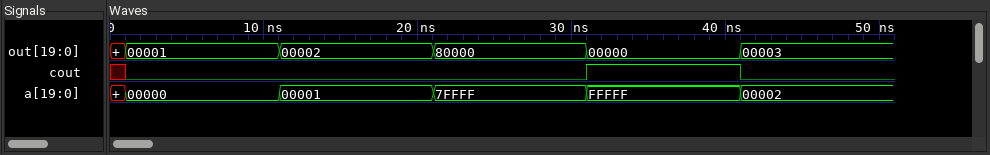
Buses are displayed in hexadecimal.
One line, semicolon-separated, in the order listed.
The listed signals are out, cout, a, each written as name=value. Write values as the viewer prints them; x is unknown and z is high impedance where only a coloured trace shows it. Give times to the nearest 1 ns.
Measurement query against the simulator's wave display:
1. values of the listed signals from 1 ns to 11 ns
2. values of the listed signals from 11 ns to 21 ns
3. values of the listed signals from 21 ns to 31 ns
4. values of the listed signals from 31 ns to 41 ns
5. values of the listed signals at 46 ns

out=00001, cout=0, a=00000; out=00002, cout=0, a=00001; out=80000, cout=0, a=7FFFF; out=00000, cout=1, a=FFFFF; out=00003, cout=0, a=00002
